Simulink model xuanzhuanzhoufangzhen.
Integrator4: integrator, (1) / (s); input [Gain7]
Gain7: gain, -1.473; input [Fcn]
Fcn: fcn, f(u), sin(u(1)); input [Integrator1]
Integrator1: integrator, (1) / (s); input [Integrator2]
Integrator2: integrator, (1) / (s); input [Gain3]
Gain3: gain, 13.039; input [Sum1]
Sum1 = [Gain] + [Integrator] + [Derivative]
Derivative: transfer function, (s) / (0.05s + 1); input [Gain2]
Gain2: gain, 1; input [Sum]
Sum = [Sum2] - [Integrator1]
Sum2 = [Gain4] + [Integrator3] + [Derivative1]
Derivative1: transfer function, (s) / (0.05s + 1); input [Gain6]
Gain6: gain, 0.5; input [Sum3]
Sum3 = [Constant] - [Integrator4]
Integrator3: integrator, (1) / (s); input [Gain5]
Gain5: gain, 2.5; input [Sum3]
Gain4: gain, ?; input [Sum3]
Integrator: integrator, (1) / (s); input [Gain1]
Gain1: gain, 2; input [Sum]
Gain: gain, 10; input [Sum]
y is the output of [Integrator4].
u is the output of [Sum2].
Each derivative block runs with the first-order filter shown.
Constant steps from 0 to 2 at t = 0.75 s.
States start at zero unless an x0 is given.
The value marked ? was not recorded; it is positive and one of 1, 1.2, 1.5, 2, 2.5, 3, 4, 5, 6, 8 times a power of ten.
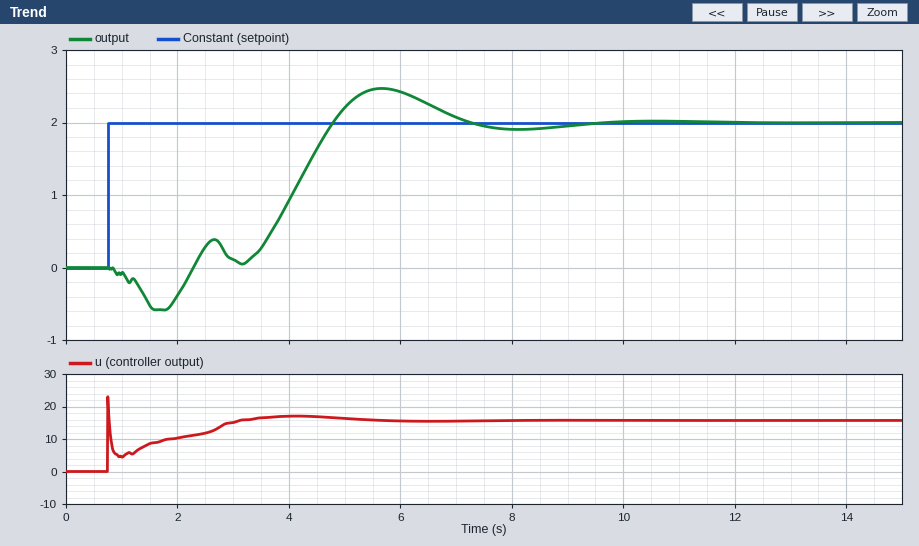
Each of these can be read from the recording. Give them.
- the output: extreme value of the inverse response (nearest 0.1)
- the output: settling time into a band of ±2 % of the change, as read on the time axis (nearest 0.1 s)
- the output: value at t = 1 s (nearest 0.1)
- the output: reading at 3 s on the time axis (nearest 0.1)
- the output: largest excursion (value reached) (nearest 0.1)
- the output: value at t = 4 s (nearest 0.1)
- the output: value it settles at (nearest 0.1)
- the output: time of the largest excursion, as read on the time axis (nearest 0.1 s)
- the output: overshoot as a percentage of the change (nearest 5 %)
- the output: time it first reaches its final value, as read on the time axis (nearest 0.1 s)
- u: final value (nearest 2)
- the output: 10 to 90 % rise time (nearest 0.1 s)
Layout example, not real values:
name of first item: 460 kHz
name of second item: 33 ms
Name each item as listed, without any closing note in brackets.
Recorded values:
the output: extreme value of the inverse response: -0.6
the output: settling time into a band of ±2 % of the change, as read on the time axis: 9.1 s
the output: value at t = 1 s: -0.1
the output: reading at 3 s on the time axis: 0.1
the output: largest excursion (value reached): 2.5
the output: value at t = 4 s: 0.9
the output: value it settles at: 2.0
the output: time of the largest excursion, as read on the time axis: 5.7 s
the output: overshoot as a percentage of the change: 25 %
the output: time it first reaches its final value, as read on the time axis: 4.8 s
u: final value: 16
the output: 10 to 90 % rise time: 2.2 s
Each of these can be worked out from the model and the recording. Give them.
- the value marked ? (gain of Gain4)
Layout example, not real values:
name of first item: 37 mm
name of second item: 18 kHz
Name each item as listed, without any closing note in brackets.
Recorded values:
the value marked ?: 1.5
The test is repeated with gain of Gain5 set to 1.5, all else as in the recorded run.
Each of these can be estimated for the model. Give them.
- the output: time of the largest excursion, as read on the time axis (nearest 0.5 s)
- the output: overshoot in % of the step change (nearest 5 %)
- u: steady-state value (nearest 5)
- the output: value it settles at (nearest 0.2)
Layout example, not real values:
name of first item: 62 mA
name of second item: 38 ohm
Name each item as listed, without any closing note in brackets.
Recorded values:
the output: time of the largest excursion, as read on the time axis: 4.0 s
the output: overshoot in % of the step change: 20 %
u: steady-state value: 5
the output: value it settles at: 2.0
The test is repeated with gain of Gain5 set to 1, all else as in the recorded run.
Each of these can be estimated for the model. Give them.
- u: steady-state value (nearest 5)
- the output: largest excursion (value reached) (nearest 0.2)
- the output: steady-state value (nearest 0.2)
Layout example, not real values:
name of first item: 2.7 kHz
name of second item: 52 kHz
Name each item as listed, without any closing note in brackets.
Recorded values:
u: steady-state value: 5
the output: largest excursion (value reached): 2.2
the output: steady-state value: 2.0
